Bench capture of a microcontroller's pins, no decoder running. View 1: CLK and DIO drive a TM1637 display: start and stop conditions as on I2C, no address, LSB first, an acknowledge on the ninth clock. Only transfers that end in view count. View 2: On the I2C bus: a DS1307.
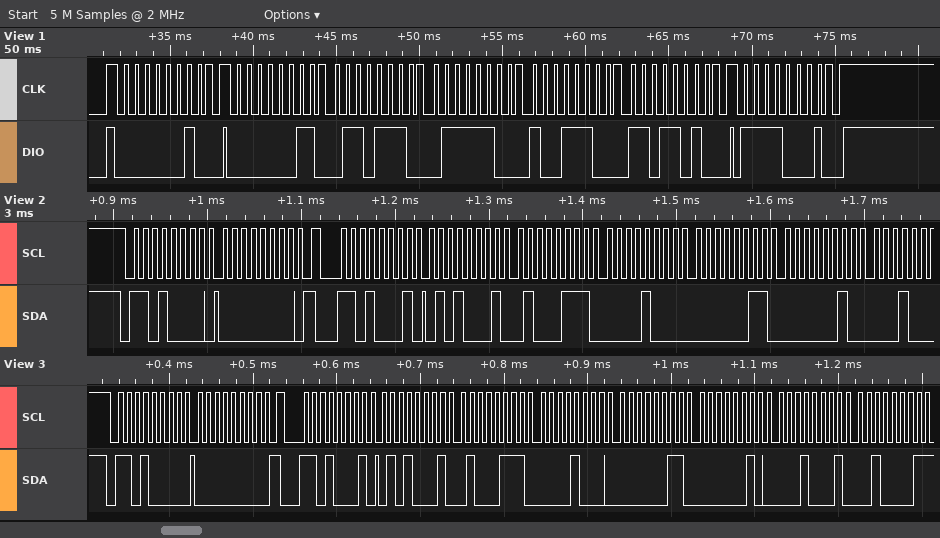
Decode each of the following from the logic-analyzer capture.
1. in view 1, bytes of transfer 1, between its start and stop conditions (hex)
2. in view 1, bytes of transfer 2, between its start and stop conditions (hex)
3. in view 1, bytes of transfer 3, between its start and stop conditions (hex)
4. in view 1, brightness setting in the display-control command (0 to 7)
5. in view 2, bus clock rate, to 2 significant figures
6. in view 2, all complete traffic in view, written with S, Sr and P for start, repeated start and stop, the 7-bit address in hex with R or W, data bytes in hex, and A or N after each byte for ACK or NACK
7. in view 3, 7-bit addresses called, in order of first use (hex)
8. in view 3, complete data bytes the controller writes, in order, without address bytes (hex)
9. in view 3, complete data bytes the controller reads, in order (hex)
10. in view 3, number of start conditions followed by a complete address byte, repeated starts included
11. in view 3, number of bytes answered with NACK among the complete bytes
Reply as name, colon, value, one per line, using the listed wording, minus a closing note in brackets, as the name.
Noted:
in view 1, bytes of transfer 1, between its start and stop conditions: 40
in view 1, bytes of transfer 2, between its start and stop conditions: C0 76 3E 39 5B
in view 1, bytes of transfer 3, between its start and stop conditions: 8F
in view 1, brightness setting in the display-control command: 7
in view 2, bus clock rate, to 2 significant figures: 100 kHz
in view 2, all complete traffic in view, written with S, Sr and P for start, repeated start and stop, the 7-bit address in hex with R or W, data bytes in hex, and A or N after each byte for ACK or NACK: S 68W A 00 A Sr 68R A 51 A 47 A 08 A 03 A 02 A
in view 3, 7-bit addresses called, in order of first use: 0x68
in view 3, complete data bytes the controller writes, in order, without address bytes: 00
in view 3, complete data bytes the controller reads, in order: 51 47 08 03 02 11 21
in view 3, number of start conditions followed by a complete address byte, repeated starts included: 2
in view 3, number of bytes answered with NACK among the complete bytes: 1
